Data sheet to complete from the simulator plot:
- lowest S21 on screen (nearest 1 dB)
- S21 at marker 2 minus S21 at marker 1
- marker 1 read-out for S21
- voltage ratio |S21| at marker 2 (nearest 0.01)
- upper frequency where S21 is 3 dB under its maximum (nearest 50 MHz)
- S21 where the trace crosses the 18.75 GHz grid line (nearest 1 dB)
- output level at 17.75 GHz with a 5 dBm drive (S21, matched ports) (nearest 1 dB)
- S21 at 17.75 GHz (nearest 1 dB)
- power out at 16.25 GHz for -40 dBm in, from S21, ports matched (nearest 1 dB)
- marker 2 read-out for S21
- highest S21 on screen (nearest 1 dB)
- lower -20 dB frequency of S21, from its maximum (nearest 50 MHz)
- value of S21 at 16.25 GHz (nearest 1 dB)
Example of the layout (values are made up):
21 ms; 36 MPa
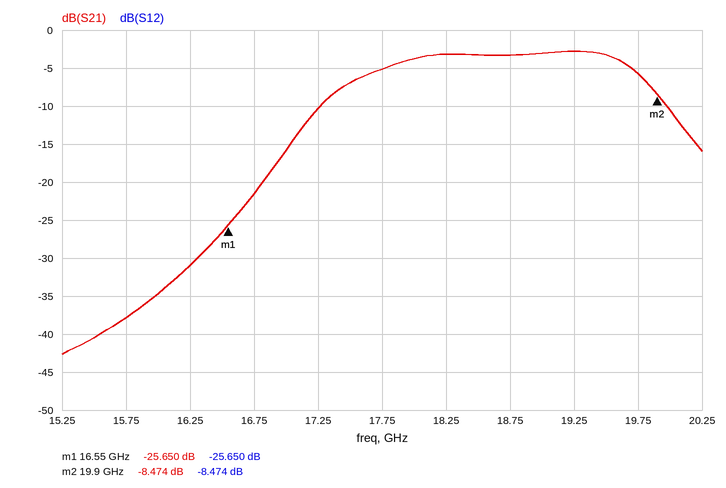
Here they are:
-43 dB; 17.176 dB; -25.650 dB; 0.38; 19.75 GHz; -3 dB; 0 dBm; -5 dB; -71 dBm; -8.474 dB; -3 dB; 16.70 GHz; -31 dB
